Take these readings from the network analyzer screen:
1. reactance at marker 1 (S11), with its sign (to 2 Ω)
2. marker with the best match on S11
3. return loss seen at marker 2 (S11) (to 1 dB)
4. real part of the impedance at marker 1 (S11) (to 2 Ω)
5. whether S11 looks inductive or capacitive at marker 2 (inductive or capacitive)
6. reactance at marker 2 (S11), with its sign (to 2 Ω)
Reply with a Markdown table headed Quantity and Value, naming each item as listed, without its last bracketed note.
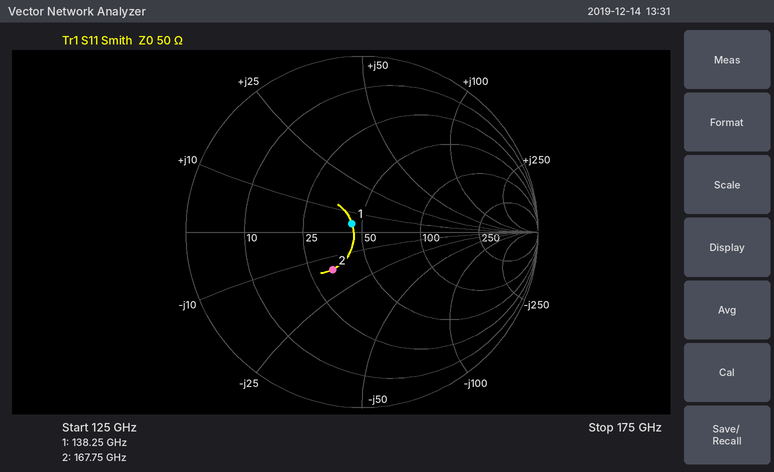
| Quantity | Value |
|---|---|
| reactance at marker 1 (S11), with its sign | +4 Ω |
| marker with the best match on S11 | marker 1 |
| return loss seen at marker 2 (S11) | 11 dB |
| real part of the impedance at marker 1 (S11) | 44 Ω |
| whether S11 looks inductive or capacitive at marker 2 | capacitive |
| reactance at marker 2 (S11), with its sign | -16 Ω |
